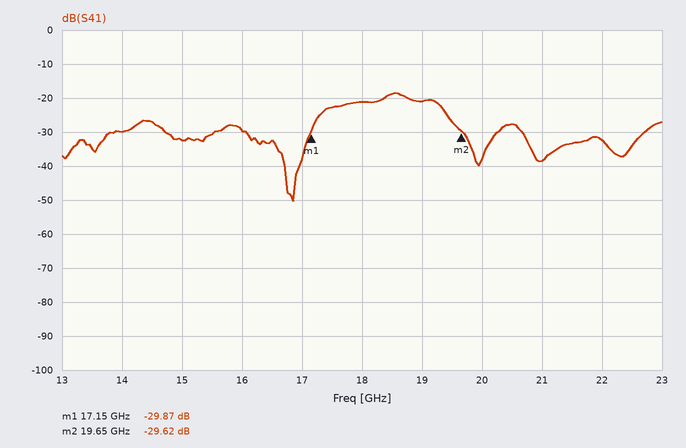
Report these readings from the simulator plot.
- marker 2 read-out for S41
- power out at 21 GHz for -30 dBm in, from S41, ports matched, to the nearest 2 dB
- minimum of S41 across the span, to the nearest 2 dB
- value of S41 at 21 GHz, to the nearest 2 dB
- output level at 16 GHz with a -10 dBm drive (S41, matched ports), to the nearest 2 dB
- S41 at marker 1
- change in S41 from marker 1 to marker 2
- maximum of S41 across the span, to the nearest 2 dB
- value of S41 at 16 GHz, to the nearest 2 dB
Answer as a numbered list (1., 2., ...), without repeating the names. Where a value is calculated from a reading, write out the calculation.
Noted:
1. -29.62 dB
2. -30 dBm + (-38 dB) = -68 dBm
3. -50 dB
4. -38 dB
5. -10 dBm + (-30 dB) = -40 dBm
6. -29.87 dB
7. -29.62 − (-29.87) = 0.25 dB
8. -18 dB
9. -30 dB
